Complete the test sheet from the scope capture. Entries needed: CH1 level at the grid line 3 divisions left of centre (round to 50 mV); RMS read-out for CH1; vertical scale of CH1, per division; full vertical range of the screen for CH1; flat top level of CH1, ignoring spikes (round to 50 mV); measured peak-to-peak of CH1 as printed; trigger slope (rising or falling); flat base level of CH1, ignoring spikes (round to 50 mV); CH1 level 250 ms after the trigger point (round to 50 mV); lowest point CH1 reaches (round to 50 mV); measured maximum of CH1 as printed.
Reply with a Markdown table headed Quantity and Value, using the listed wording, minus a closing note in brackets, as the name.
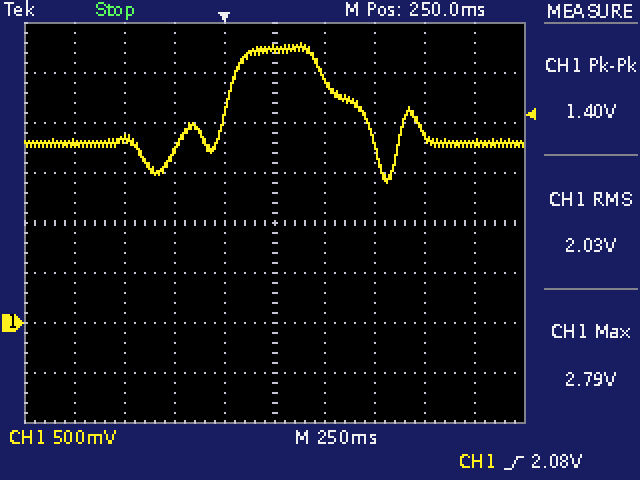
| Quantity | Value |
|---|---|
| CH1 level at the grid line 3 divisions left of centre | 1.85 V |
| RMS read-out for CH1 | 2.03 V |
| vertical scale of CH1, per division | 500 mV |
| full vertical range of the screen for CH1 | 4 V |
| flat top level of CH1, ignoring spikes | 2.75 V |
| measured peak-to-peak of CH1 as printed | 1.40 V |
| trigger slope | rising |
| flat base level of CH1, ignoring spikes | 1.80 V |
| CH1 level 250 ms after the trigger point | 2.75 V |
| lowest point CH1 reaches | 1.40 V |
| measured maximum of CH1 as printed | 2.79 V |
